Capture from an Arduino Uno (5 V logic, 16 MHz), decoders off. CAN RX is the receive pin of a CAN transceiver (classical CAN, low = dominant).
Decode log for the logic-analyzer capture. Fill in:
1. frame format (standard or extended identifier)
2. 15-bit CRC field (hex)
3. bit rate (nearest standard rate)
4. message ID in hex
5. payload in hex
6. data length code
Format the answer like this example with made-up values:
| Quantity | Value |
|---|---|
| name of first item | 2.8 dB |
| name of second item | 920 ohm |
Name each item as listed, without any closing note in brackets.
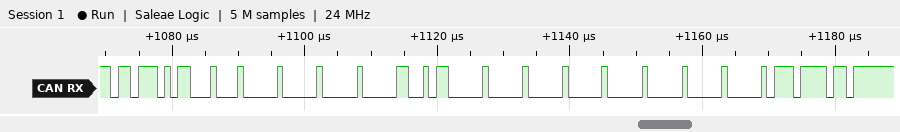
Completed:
| Quantity | Value |
|---|---|
| frame format | standard |
| 15-bit CRC field | 0x03BD |
| bit rate | 1000 kbit/s |
| message ID in hex | 0x6EB |
| payload in hex | 80 00 04 B0 00 00 00 00 |
| data length code | 8 |
